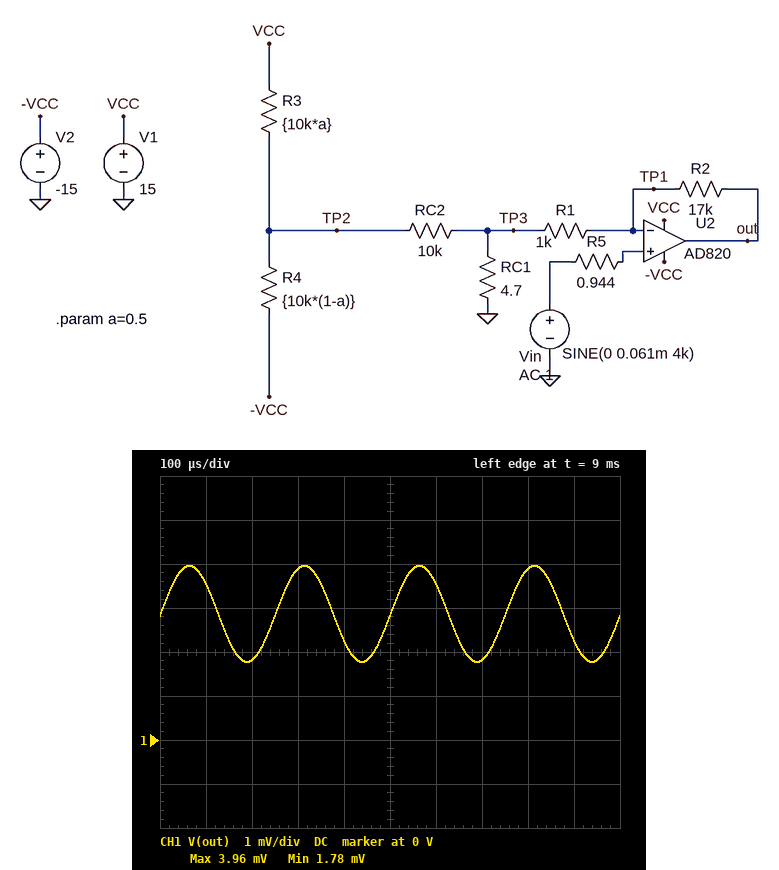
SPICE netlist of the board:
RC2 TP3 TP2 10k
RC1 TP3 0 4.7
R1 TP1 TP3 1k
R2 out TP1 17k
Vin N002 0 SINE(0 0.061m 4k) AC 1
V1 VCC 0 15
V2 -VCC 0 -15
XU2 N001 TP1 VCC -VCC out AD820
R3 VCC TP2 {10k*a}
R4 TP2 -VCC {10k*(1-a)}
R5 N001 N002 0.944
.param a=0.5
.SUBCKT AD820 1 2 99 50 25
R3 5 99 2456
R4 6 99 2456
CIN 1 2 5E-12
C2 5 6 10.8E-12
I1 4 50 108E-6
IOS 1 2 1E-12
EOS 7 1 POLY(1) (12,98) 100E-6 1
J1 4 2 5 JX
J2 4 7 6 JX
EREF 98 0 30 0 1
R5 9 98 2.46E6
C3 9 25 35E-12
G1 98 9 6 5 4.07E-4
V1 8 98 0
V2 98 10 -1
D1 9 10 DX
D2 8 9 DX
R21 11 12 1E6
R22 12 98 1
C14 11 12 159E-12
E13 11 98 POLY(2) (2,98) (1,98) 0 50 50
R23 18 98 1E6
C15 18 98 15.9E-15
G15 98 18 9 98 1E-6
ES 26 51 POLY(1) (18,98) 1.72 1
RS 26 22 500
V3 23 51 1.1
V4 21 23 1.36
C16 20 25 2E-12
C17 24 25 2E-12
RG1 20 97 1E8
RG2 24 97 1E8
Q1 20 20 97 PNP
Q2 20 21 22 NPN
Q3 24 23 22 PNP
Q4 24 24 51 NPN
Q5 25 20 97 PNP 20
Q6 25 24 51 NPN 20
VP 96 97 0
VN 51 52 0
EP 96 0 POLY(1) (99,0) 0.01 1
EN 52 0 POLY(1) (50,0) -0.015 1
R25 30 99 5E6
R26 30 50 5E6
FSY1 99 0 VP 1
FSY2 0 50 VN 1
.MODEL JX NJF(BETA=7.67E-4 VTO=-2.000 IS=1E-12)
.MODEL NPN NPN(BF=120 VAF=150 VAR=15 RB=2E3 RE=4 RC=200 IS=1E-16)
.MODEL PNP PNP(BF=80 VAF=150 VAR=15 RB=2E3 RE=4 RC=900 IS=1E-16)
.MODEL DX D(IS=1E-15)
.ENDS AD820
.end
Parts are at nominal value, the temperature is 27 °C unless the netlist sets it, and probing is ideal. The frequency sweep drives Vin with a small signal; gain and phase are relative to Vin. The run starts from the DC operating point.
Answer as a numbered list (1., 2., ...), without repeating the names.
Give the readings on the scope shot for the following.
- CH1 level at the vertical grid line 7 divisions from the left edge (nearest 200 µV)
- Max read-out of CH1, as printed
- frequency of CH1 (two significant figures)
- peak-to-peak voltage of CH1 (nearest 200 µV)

1. 1.8 mV
2. 3.96 mV
3. 4.0 kHz
4. 2.2 mV
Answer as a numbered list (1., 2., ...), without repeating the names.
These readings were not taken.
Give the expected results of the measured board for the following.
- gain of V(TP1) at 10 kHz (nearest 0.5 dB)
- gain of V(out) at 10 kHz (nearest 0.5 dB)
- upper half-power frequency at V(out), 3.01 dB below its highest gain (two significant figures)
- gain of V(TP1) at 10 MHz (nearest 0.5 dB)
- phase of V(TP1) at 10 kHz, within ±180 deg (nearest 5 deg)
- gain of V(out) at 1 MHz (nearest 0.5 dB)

1. 0 dB
2. 25.0 dB
3. 110 kHz
4. -11.0 dB
5. -5 deg
6. 5.0 dB
